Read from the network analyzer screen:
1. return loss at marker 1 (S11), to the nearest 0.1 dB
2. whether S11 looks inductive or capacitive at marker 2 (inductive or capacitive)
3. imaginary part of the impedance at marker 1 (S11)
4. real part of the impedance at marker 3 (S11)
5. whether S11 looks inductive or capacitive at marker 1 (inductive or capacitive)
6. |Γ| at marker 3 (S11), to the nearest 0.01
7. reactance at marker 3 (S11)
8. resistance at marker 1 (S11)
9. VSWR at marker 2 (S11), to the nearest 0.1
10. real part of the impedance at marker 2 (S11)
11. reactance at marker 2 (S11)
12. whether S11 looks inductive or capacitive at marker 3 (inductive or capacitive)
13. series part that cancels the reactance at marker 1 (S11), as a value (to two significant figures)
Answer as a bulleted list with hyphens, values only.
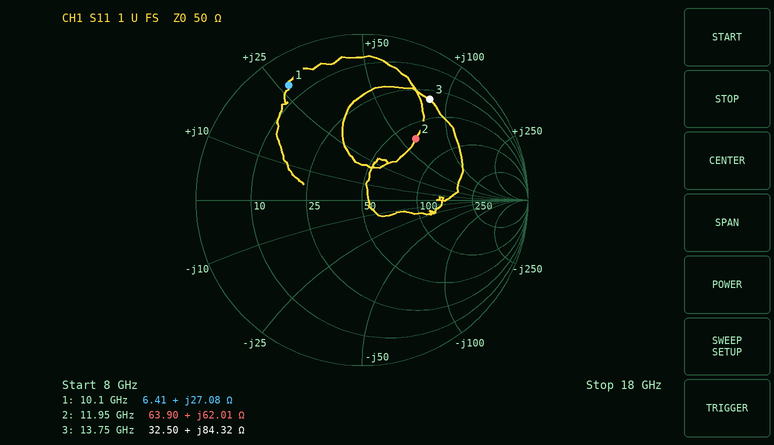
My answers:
- 1.7 dB
- inductive
- +27.08 Ω
- 32.50 Ω
- inductive
- 0.73
- +84.32 Ω
- 6.41 Ω
- 2.9
- 63.90 Ω
- +62.01 Ω
- inductive
- 580 fF
